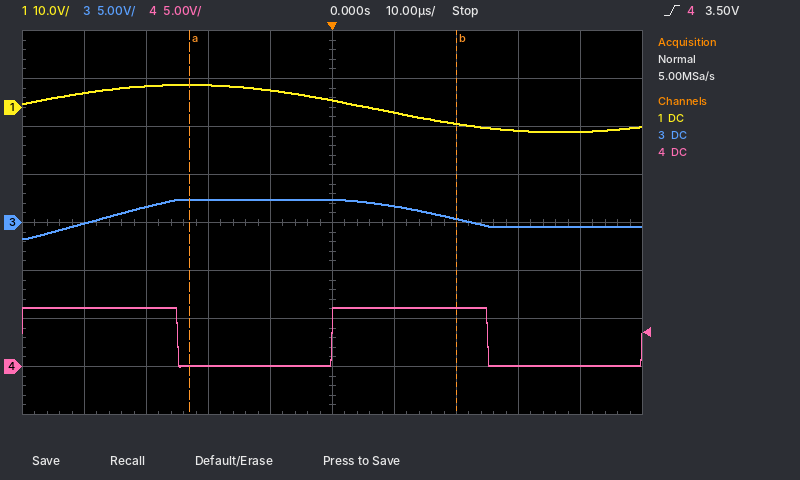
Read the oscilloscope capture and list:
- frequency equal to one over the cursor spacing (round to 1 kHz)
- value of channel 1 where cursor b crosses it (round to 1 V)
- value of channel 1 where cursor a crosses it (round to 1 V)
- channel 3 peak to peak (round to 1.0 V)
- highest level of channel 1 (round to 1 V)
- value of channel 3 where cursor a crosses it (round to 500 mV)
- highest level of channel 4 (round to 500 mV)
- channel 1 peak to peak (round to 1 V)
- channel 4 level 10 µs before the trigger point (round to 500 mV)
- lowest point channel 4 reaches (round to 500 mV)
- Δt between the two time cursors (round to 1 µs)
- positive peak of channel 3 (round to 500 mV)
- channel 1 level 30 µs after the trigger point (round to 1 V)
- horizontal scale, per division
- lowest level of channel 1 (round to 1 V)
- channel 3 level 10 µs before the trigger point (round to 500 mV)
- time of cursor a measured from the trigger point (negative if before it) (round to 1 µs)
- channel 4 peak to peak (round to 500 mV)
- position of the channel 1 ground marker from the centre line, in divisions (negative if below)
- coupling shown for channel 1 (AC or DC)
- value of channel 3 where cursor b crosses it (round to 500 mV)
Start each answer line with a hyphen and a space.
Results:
- 23 kHz
- -3 V
- 5 V
- 4.0 V
- 5 V
- 2.5 V
- 6.0 V
- 10 V
- 0.0 V
- 0.0 V
- 43 µs
- 2.5 V
- -5 V
- 10 µs
- -5 V
- 2.5 V
- -23 µs
- 6.0 V
- +2.4 div
- DC
- 500 mV
